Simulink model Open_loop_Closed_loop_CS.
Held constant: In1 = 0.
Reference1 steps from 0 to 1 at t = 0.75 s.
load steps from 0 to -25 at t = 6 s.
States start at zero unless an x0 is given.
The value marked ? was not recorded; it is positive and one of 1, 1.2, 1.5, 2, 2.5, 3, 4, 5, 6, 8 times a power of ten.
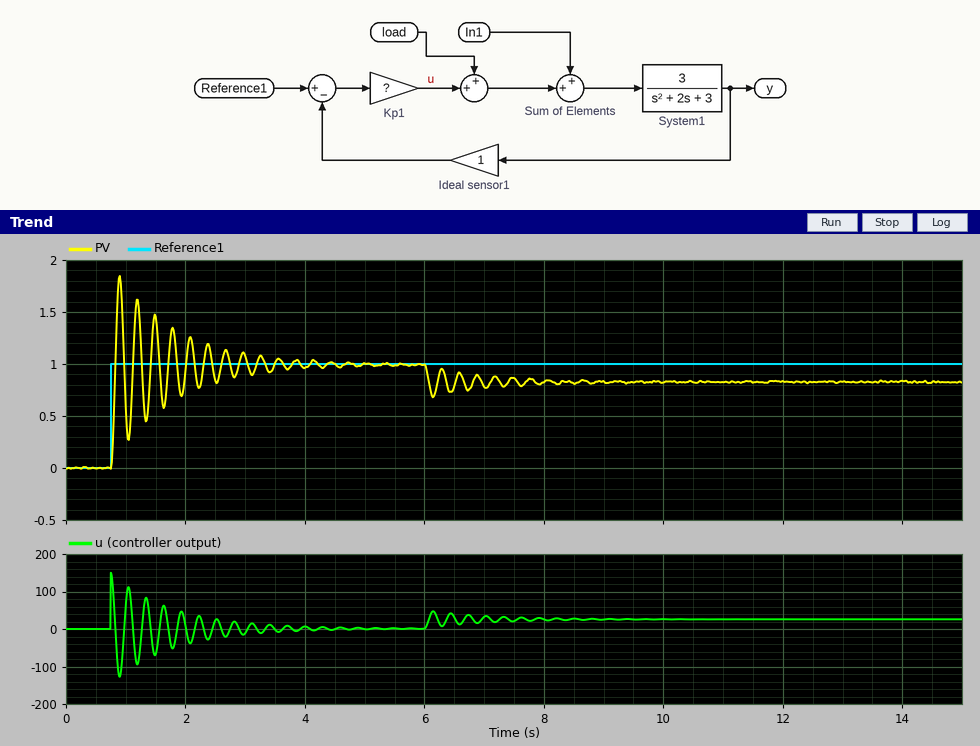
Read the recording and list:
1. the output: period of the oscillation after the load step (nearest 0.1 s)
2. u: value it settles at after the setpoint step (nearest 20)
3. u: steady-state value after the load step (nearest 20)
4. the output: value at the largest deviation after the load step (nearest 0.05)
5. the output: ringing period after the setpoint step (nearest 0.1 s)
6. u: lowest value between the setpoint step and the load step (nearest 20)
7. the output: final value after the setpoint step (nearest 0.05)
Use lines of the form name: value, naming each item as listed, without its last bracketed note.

the output: period of the oscillation after the load step: 0.3 s
u: value it settles at after the setpoint step: 0
u: steady-state value after the load step: 20
the output: value at the largest deviation after the load step: 0.70
the output: ringing period after the setpoint step: 0.3 s
u: lowest value between the setpoint step and the load step: -120
the output: final value after the setpoint step: 1.00
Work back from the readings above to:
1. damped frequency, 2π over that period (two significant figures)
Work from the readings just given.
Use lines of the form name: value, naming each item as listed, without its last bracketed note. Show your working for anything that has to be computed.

damped frequency, 2π over that period: 2π / 0.3 = 21 rad/s
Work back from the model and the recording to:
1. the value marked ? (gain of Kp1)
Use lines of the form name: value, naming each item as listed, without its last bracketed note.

the value marked ?: 150
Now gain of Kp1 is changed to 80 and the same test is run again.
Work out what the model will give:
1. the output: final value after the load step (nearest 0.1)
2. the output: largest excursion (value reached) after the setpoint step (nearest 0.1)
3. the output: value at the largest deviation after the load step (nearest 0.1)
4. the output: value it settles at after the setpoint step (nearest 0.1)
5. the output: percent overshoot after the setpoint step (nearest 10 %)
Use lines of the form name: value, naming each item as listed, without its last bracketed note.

the output: final value after the load step: 0.7
the output: largest excursion (value reached) after the setpoint step: 1.8
the output: value at the largest deviation after the load step: 0.4
the output: value it settles at after the setpoint step: 1.0
the output: percent overshoot after the setpoint step: 80 %
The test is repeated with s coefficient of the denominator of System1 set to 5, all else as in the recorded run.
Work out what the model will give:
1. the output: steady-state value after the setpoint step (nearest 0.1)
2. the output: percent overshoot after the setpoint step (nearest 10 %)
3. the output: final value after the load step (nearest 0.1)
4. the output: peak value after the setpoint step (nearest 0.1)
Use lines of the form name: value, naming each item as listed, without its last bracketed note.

the output: steady-state value after the setpoint step: 1.0
the output: percent overshoot after the setpoint step: 70 %
the output: final value after the load step: 0.8
the output: peak value after the setpoint step: 1.7
